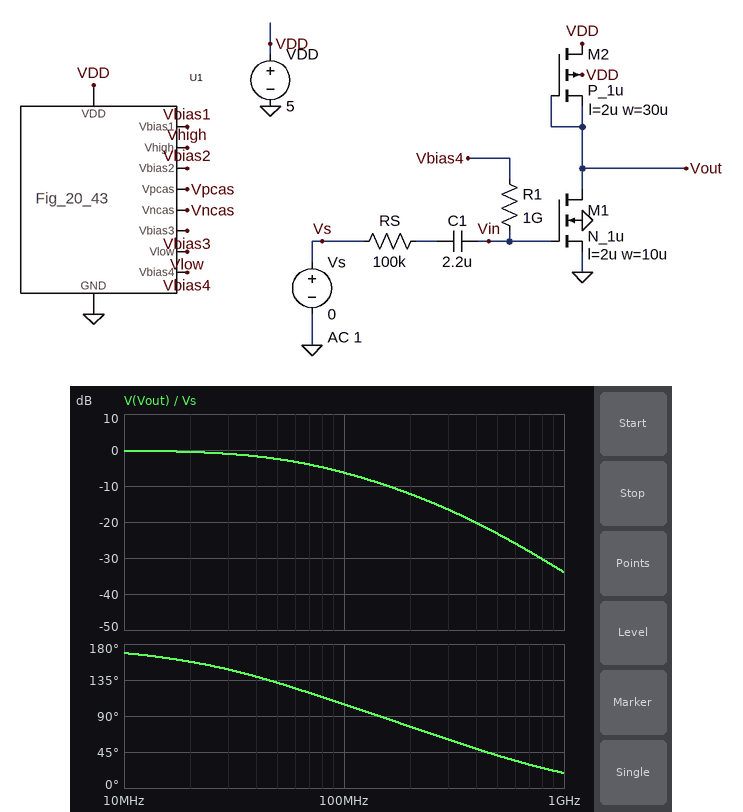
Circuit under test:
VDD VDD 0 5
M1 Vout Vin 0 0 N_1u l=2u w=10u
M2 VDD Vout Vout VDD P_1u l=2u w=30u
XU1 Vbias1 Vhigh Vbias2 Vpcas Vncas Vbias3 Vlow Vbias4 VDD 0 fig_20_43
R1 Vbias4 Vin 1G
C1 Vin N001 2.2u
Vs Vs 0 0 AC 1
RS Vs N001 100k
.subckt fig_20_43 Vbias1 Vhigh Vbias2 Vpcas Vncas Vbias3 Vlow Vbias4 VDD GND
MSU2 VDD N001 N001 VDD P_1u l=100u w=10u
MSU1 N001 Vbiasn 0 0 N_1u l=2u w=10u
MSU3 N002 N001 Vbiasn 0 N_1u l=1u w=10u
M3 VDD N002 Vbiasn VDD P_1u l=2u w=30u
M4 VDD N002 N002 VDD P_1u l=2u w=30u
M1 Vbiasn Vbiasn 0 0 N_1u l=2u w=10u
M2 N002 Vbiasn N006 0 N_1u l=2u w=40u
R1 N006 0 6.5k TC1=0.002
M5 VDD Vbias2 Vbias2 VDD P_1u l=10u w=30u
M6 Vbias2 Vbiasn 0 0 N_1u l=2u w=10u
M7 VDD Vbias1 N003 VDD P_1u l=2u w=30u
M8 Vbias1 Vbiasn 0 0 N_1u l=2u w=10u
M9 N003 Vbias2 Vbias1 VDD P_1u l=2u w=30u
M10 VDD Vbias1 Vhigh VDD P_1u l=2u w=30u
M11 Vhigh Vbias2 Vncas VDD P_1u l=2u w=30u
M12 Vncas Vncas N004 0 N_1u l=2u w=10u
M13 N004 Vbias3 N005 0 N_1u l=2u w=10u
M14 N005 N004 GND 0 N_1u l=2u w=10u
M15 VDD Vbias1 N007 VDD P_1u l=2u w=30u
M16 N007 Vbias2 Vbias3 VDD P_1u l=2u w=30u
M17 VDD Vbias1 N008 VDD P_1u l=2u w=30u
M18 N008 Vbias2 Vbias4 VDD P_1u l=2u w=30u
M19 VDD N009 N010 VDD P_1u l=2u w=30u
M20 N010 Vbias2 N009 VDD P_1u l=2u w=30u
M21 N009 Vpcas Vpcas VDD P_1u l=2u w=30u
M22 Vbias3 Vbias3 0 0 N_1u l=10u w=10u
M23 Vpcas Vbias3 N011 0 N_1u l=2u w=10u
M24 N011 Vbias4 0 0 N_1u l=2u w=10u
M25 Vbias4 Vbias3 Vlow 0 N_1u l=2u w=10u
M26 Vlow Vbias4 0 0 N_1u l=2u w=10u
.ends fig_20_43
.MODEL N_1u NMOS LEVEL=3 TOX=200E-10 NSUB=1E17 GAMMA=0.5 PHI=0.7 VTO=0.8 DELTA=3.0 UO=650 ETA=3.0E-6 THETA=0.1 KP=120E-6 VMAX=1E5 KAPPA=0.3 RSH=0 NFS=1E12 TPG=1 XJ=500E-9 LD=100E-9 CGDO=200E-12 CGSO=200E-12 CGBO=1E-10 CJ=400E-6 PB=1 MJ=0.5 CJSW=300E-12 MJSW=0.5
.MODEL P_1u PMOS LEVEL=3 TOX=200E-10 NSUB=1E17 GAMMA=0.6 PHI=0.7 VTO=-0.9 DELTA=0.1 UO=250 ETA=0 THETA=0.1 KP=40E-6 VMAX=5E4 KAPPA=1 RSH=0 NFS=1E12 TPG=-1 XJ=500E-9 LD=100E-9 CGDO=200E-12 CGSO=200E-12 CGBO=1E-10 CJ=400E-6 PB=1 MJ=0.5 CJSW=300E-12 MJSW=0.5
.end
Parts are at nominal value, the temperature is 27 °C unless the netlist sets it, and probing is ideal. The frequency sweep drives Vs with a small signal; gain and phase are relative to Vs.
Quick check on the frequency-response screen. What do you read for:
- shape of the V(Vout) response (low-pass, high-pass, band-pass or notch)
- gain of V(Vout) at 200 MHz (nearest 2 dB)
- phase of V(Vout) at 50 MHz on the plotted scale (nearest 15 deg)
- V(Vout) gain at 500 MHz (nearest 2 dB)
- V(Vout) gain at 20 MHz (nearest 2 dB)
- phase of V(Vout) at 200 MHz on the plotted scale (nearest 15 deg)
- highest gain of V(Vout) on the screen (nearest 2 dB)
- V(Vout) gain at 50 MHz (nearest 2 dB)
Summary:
low-pass
-12 dB
135 deg
-24 dB
0 dB
75 deg
0 dB
-2 dB
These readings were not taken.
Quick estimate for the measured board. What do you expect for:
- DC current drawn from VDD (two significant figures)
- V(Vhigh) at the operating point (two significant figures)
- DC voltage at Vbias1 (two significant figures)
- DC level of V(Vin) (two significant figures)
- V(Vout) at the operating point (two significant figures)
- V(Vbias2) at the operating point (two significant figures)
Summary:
210 µA
4.7 V
3.8 V
1.1 V
3.8 V
3.4 V
